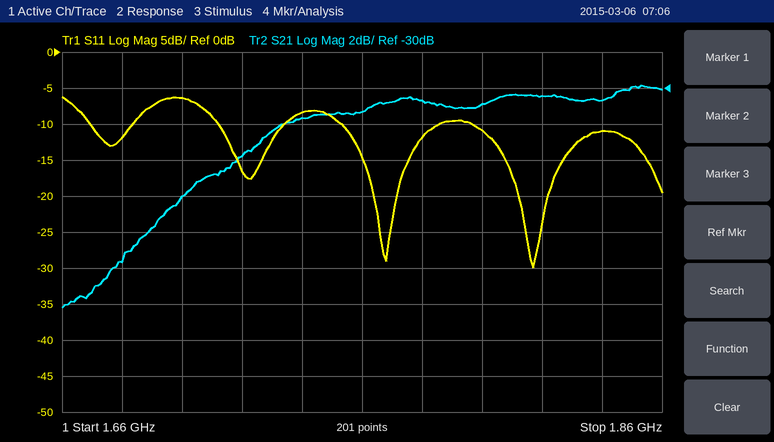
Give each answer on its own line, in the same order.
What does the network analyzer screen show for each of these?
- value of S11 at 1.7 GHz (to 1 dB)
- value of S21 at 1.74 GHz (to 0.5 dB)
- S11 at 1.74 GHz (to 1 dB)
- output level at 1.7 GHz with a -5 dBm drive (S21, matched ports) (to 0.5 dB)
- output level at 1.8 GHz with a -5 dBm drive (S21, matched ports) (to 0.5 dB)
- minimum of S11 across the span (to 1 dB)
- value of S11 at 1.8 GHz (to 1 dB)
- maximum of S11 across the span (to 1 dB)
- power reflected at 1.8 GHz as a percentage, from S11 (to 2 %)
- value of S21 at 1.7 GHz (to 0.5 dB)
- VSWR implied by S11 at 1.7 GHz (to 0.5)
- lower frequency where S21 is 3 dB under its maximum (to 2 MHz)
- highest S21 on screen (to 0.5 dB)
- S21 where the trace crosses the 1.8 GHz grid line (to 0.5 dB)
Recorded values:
-6 dB
-31.5 dB
-8 dB
-41.0 dBm
-36.0 dBm
-30 dB
-11 dB
-6 dB
8 %
-36.0 dB
3.0
1.726 GHz
-30.0 dB
-31.0 dB
